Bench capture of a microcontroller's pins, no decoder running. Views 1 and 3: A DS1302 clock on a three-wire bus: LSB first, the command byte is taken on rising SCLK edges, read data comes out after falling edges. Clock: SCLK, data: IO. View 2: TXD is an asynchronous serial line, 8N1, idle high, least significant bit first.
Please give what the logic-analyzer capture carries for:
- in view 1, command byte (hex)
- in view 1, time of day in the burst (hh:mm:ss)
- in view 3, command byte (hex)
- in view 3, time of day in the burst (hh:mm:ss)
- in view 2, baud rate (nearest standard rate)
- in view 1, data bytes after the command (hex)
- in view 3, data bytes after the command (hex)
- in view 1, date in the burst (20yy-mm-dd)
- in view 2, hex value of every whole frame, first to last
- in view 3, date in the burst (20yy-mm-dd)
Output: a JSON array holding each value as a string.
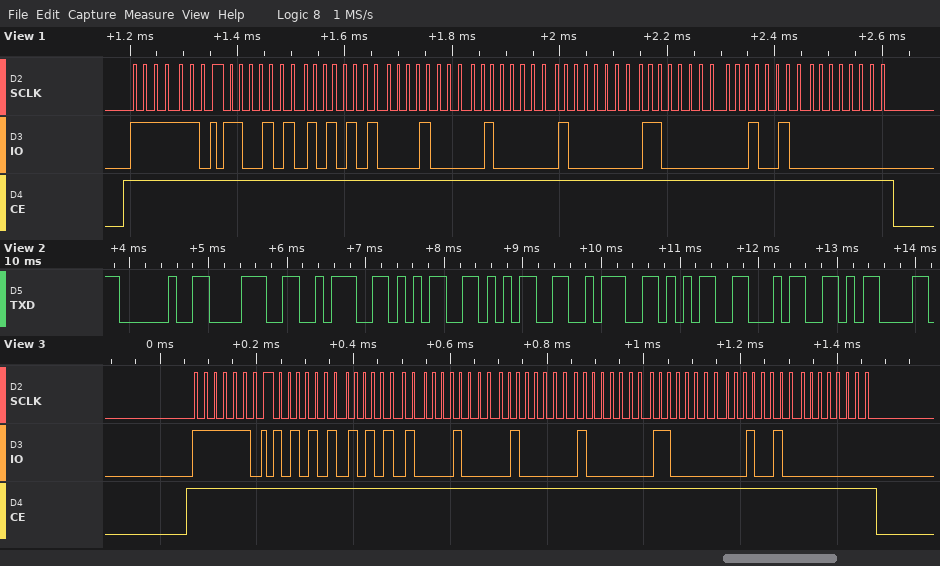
["0xBF", "08:55:53", "0xBF", "08:55:55", "9600 baud", "53 55 08 02 01 03 24 00", "55 55 08 02 01 03 24 00", "2024-01-02", "20 38 3A 35 35 3A 35 34 0D", "2024-01-02"]
